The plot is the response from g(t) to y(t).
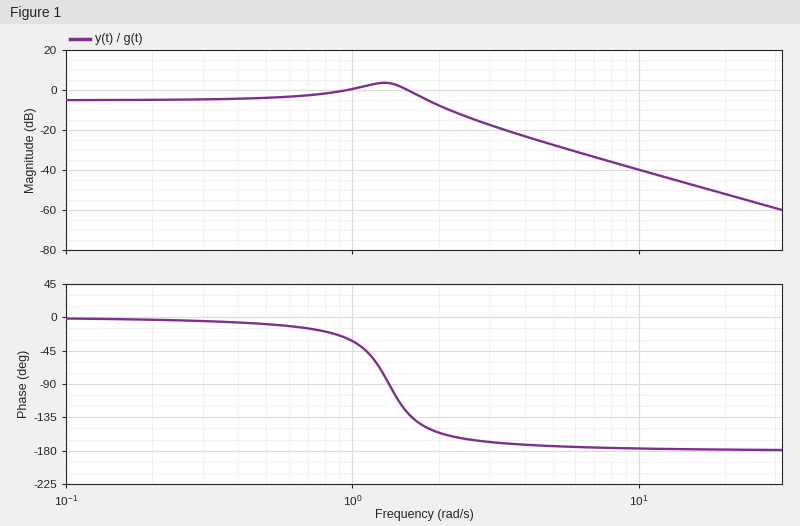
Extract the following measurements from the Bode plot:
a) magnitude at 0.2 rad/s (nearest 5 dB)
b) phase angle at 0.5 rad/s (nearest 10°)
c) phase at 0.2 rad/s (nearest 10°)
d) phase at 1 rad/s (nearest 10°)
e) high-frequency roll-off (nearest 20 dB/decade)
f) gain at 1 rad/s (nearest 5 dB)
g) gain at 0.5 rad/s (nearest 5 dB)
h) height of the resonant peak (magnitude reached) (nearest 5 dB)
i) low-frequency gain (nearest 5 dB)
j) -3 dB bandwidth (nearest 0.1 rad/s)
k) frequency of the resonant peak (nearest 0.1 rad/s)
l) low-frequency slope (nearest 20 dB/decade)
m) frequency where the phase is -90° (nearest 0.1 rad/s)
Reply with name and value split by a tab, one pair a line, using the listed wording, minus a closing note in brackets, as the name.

magnitude at 0.2 rad/s	-5 dB
phase angle at 0.5 rad/s	-10°
phase at 0.2 rad/s	0°
phase at 1 rad/s	-30°
high-frequency roll-off	-40 dB/decade
gain at 1 rad/s	0 dB
gain at 0.5 rad/s	-5 dB
height of the resonant peak (magnitude reached)	5 dB
low-frequency gain	-5 dB
-3 dB bandwidth	2.0 rad/s
frequency of the resonant peak	1.3 rad/s
low-frequency slope	0 dB/decade
frequency where the phase is -90°	1.3 rad/s
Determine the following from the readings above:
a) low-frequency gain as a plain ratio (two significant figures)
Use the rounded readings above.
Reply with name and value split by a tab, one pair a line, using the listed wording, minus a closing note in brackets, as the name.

low-frequency gain as a plain ratio	0.56
